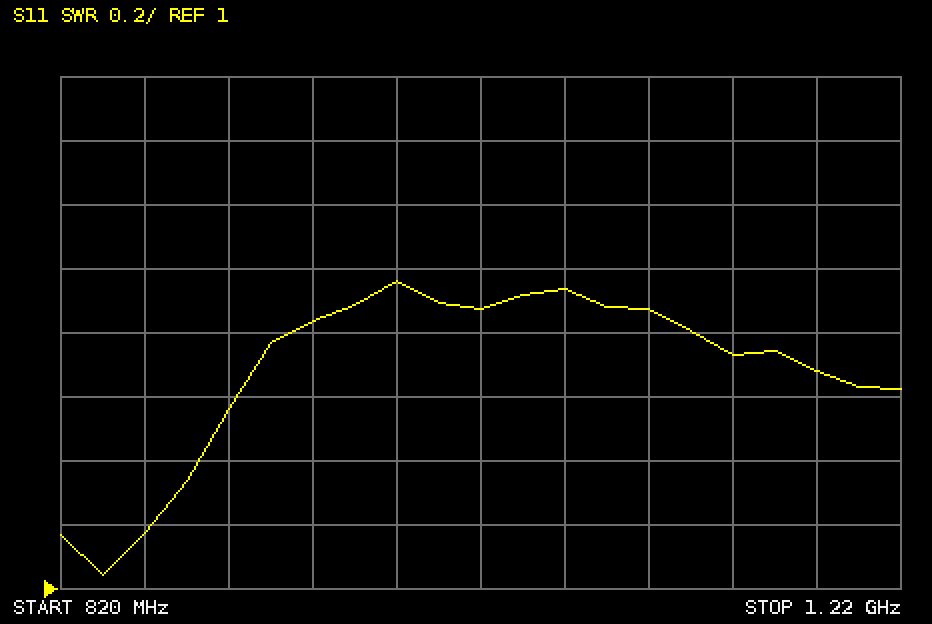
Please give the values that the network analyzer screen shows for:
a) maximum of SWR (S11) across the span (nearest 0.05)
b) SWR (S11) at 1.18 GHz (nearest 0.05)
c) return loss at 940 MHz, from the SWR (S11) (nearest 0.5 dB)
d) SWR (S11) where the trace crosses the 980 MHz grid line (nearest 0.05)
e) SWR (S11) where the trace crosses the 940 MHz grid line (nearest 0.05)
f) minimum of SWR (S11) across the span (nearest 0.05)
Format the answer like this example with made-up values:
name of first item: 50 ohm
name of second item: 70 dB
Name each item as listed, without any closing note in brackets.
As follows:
maximum of SWR (S11) across the span: 1.95
SWR (S11) at 1.18 GHz: 1.70
return loss at 940 MHz, from the SWR (S11): 10.5 dB
SWR (S11) where the trace crosses the 980 MHz grid line: 1.95
SWR (S11) where the trace crosses the 940 MHz grid line: 1.85
minimum of SWR (S11) across the span: 1.05
